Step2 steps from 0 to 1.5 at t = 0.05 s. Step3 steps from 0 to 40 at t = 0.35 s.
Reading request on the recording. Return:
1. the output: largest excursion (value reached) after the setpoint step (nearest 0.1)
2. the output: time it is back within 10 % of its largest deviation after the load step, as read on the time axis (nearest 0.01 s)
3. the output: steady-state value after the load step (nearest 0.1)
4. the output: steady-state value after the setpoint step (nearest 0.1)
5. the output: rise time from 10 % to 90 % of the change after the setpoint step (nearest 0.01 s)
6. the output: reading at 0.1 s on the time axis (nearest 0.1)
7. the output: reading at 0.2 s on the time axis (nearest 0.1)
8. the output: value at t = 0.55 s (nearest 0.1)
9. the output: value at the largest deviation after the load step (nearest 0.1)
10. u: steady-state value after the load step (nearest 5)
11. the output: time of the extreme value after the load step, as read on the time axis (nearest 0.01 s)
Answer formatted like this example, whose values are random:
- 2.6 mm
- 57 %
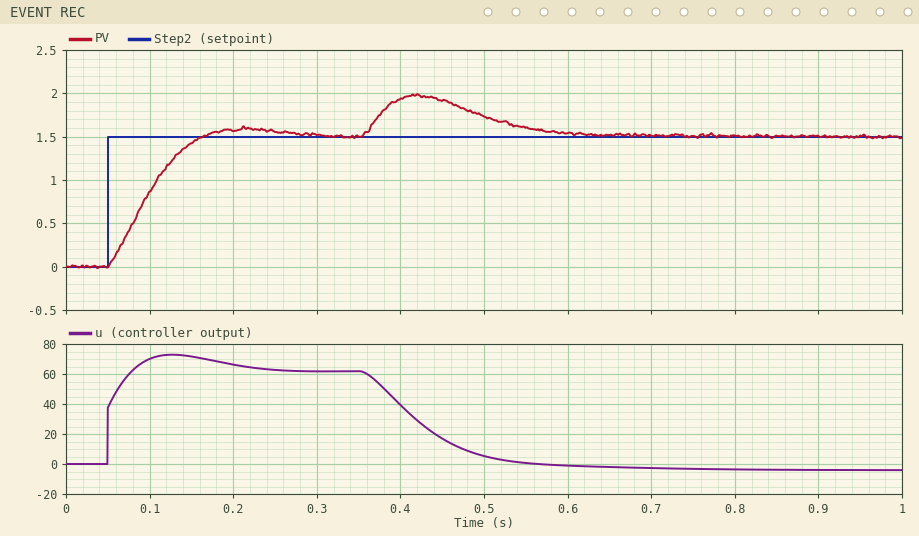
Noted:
- 1.6
- 0.59 s
- 1.5
- 1.5
- 0.08 s
- 0.9
- 1.6
- 1.6
- 2.0
- -5
- 0.42 s
